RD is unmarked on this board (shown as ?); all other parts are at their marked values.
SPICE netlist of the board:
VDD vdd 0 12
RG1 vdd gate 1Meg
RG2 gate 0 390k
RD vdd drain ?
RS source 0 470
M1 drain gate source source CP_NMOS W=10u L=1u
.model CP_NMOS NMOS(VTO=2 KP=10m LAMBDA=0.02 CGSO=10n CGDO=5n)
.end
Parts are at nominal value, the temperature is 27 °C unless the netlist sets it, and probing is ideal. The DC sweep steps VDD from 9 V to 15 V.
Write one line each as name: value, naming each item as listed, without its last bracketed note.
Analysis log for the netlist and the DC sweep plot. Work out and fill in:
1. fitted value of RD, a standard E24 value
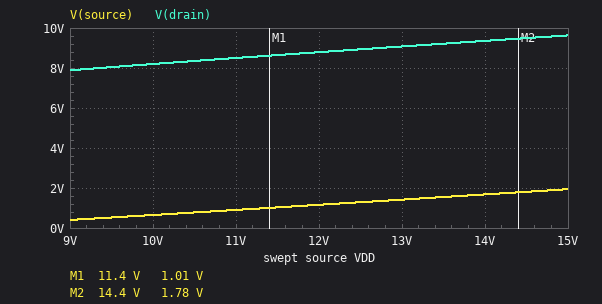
fitted value of RD, a standard E24 value: 1.3 kΩ
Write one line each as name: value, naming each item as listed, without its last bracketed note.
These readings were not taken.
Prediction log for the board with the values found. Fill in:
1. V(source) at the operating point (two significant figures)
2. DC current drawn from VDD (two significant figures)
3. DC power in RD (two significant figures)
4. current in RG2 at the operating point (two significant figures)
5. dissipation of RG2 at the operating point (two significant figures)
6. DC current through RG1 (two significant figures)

V(source) at the operating point: 1.2 V
DC current drawn from VDD: 2.5 mA
DC power in RD: 7.9 mW
current in RG2 at the operating point: 8.6 µA
dissipation of RG2 at the operating point: 29 µW
DC current through RG1: 8.6 µA
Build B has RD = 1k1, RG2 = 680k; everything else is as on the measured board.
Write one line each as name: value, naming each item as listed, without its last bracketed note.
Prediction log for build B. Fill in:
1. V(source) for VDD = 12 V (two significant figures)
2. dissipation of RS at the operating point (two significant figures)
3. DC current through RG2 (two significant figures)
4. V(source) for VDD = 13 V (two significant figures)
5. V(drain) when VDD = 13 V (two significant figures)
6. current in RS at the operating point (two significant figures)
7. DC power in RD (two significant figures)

V(source) for VDD = 12 V: 2.5 V
dissipation of RS at the operating point: 14 mW
DC current through RG2: 7.1 µA
V(source) for VDD = 13 V: 2.9 V
V(drain) when VDD = 13 V: 6.2 V
current in RS at the operating point: 5.4 mA
DC power in RD: 32 mW
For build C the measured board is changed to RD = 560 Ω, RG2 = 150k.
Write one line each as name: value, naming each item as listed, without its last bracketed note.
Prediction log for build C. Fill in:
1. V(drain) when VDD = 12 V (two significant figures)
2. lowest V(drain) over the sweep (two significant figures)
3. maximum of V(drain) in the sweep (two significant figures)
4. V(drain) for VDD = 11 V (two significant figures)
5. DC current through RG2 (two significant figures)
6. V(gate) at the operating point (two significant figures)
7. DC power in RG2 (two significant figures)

V(drain) when VDD = 12 V: 12 V
lowest V(drain) over the sweep: 9.0 V
maximum of V(drain) in the sweep: 15 V
V(drain) for VDD = 11 V: 11 V
DC current through RG2: 10 µA
V(gate) at the operating point: 1.6 V
DC power in RG2: 16 µW
